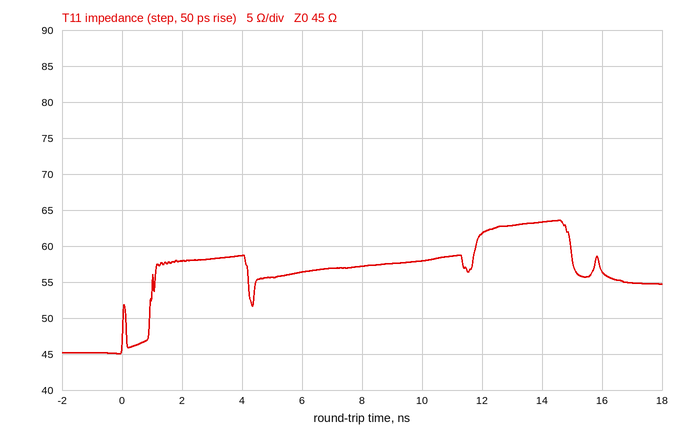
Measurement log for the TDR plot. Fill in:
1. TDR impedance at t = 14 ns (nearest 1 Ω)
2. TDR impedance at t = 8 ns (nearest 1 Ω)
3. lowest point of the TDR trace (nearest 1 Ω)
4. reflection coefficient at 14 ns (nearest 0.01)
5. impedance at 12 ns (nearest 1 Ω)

63 Ω
57 Ω
45 Ω
+0.17
62 Ω
